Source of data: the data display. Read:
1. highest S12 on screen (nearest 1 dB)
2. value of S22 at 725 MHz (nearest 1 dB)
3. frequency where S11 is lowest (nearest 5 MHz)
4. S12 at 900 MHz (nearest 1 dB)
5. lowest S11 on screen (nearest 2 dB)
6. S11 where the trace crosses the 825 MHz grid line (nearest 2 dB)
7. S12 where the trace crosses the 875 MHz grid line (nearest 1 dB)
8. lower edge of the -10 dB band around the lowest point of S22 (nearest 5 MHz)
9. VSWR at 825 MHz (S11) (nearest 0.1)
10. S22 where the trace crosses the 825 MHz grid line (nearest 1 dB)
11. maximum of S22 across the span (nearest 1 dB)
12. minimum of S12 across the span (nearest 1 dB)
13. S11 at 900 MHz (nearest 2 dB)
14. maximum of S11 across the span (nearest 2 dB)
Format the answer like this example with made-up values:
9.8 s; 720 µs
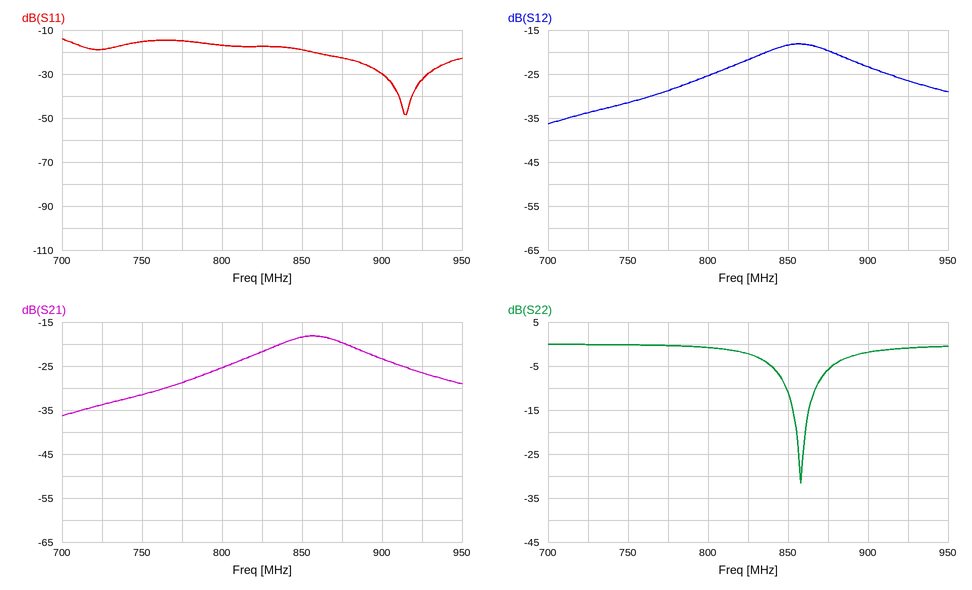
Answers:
-18 dB; 0 dB; 915 MHz; -23 dB; -48 dB; -18 dB; -20 dB; 850 MHz; 1.3; -2 dB; 0 dB; -36 dB; -30 dB; -14 dB
